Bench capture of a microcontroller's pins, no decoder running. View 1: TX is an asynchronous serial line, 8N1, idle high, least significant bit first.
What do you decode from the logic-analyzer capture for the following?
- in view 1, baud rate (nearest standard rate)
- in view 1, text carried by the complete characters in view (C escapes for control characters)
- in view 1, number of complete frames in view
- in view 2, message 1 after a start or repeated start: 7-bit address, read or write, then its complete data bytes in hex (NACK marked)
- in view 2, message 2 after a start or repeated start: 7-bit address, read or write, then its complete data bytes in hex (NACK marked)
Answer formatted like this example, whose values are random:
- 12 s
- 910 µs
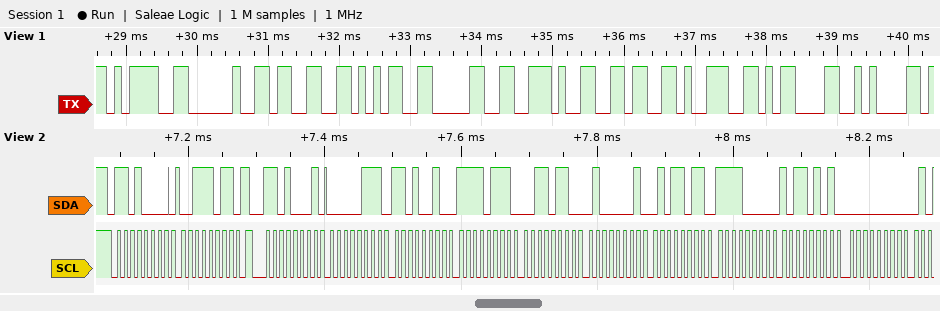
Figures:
- 9600 baud
- "= 350.69\r\n"
- 10
- 0x68 write: 3B
- 0x68 read: 07 D2 F7 36 41 5B F0 B5 00
